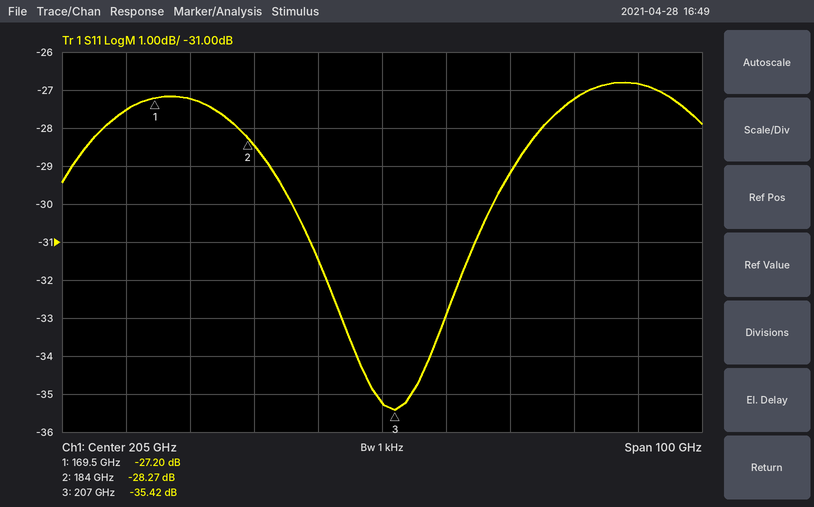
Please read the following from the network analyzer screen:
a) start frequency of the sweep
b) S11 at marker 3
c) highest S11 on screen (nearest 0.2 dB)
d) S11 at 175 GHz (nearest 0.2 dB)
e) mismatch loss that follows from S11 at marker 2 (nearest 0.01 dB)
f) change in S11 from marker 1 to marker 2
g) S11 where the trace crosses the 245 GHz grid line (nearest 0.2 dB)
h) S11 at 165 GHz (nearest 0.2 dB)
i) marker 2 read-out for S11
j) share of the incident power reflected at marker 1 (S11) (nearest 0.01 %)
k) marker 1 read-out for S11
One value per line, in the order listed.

155 GHz
-35.42 dB
-26.8 dB
-27.2 dB
0.01 dB
-1.07 dB
-26.8 dB
-27.6 dB
-28.27 dB
0.19 %
-27.20 dB
